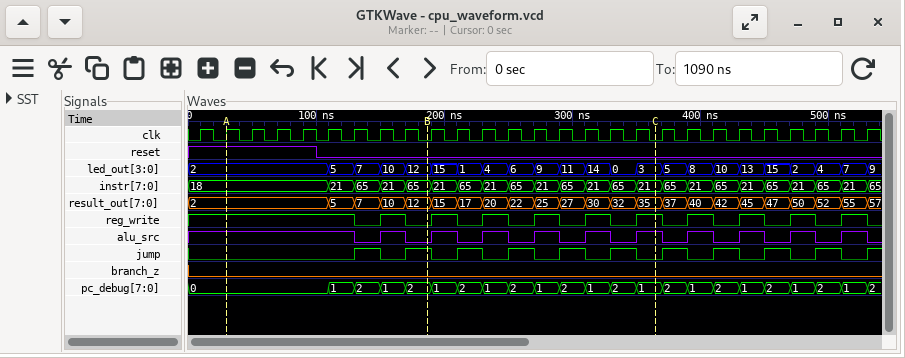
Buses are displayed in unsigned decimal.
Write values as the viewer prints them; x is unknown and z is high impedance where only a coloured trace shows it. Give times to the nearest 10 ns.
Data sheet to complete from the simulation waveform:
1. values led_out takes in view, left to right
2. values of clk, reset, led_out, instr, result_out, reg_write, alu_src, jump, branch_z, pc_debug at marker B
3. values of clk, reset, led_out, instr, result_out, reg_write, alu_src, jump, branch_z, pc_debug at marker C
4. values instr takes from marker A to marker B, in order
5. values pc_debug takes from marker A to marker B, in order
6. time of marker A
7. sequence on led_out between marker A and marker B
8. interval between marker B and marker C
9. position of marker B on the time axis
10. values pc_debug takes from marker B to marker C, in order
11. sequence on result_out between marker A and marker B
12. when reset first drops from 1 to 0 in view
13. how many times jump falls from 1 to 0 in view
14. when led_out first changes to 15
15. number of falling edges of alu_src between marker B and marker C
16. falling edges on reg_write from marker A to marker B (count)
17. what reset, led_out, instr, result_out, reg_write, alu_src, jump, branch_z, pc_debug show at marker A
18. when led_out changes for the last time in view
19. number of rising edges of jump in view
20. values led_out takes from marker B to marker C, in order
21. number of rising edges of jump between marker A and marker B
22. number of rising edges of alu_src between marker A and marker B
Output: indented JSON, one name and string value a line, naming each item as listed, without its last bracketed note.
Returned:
{
  "values led_out takes in view, left to right": "2, 5, 7, 10, 12, 15, 1, 4, 6, 9, 11, 14, 0, 3, 5, 8, 10, 13, 15, 2, 4, 7, 9",
  "values of clk, reset, led_out, instr, result_out, reg_write, alu_src, jump, branch_z, pc_debug at marker B": "clk=0, reset=0, led_out=12, instr=65, result_out=12, reg_write=0, alu_src=0, jump=1, branch_z=0, pc_debug=2",
  "values of clk, reset, led_out, instr, result_out, reg_write, alu_src, jump, branch_z, pc_debug at marker C": "clk=0, reset=0, led_out=3, instr=21, result_out=35, reg_write=1, alu_src=1, jump=0, branch_z=0, pc_debug=1",
  "values instr takes from marker A to marker B, in order": "18, 21, 65, 21, 65",
  "values pc_debug takes from marker A to marker B, in order": "0, 1, 2, 1, 2",
  "time of marker A": "30 ns",
  "sequence on led_out between marker A and marker B": "2, 5, 7, 10, 12",
  "interval between marker B and marker C": "180 ns",
  "position of marker B on the time axis": "190 ns",
  "values pc_debug takes from marker B to marker C, in order": "2, 1, 2, 1, 2, 1, 2, 1, 2, 1",
  "sequence on result_out between marker A and marker B": "2, 5, 7, 10, 12",
  "when reset first drops from 1 to 0 in view": "100 ns",
  "how many times jump falls from 1 to 0 in view": "10",
  "when led_out first changes to 15": "190 ns",
  "number of falling edges of alu_src between marker B and marker C": "4",
  "falling edges on reg_write from marker A to marker B": "2",
  "what reset, led_out, instr, result_out, reg_write, alu_src, jump, branch_z, pc_debug show at marker A": "reset=1, led_out=2, instr=18, result_out=2, reg_write=1, alu_src=1, jump=0, branch_z=0, pc_debug=0",
  "when led_out changes for the last time in view": "530 ns",
  "number of rising edges of jump in view": "11",
  "values led_out takes from marker B to marker C, in order": "12, 15, 1, 4, 6, 9, 11, 14, 0, 3",
  "number of rising edges of jump between marker A and marker B": "2",
  "number of rising edges of alu_src between marker A and marker B": "1"
}
